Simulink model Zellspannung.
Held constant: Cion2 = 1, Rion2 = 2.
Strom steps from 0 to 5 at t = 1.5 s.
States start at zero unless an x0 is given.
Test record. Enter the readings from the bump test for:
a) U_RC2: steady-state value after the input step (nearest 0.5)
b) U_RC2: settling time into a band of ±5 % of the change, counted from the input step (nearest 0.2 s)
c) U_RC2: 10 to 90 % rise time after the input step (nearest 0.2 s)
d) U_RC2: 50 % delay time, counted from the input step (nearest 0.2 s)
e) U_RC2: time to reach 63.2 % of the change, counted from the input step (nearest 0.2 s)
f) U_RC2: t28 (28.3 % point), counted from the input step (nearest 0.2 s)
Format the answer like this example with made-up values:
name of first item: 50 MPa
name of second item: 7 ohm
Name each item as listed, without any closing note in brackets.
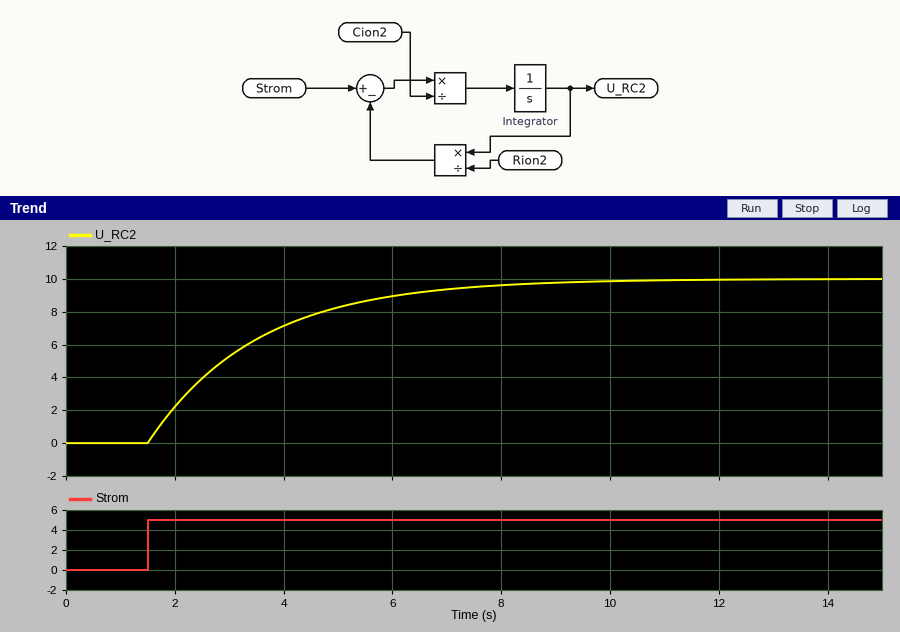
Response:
U_RC2: steady-state value after the input step: 10.0
U_RC2: settling time into a band of ±5 % of the change, counted from the input step: 6.0 s
U_RC2: 10 to 90 % rise time after the input step: 4.4 s
U_RC2: 50 % delay time, counted from the input step: 1.4 s
U_RC2: time to reach 63.2 % of the change, counted from the input step: 2.0 s
U_RC2: t28 (28.3 % point), counted from the input step: 0.6 s
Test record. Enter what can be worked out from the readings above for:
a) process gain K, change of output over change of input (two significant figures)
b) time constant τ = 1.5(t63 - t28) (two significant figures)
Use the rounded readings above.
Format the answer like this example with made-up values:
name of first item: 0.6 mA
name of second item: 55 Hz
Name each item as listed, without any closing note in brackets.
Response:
process gain K, change of output over change of input: 2.0
time constant τ = 1.5(t63 - t28): 2.1 s
